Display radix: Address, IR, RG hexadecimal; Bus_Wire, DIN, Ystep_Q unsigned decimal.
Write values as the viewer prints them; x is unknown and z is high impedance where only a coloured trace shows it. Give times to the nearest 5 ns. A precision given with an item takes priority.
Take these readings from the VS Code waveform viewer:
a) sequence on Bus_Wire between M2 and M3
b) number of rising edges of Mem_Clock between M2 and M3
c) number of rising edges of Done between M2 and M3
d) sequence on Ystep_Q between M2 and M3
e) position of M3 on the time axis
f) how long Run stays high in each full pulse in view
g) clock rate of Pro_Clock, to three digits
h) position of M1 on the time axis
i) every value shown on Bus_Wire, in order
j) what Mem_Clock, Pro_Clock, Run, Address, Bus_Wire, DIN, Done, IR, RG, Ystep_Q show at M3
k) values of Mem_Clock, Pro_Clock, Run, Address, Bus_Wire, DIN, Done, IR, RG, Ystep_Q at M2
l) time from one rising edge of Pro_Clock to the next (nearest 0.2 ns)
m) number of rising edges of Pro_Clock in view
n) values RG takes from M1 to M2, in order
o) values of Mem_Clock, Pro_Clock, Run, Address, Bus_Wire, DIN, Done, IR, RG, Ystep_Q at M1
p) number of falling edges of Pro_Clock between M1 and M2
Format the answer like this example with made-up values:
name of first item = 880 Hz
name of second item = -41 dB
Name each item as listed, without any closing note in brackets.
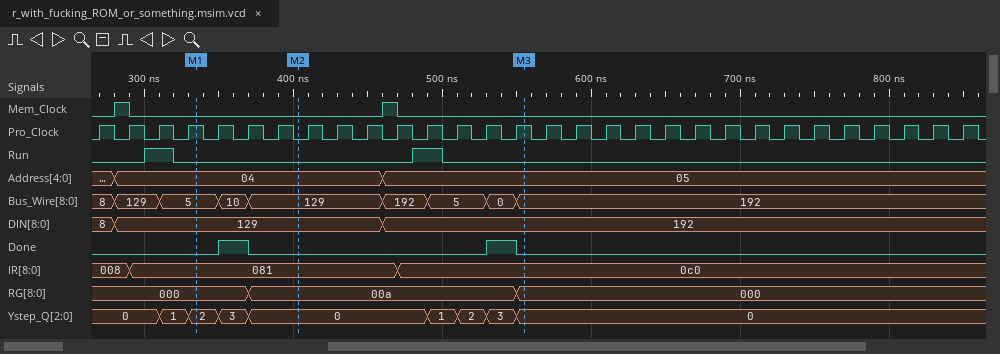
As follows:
sequence on Bus_Wire between M2 and M3 = 129, 192, 5, 0, 192
number of rising edges of Mem_Clock between M2 and M3 = 1
number of rising edges of Done between M2 and M3 = 1
sequence on Ystep_Q between M2 and M3 = 0, 1, 2, 3, 0
position of M3 on the time axis = 555 ns
how long Run stays high in each full pulse in view = 20 ns, 20 ns
clock rate of Pro_Clock, to three digits = 50.0 MHz
position of M1 on the time axis = 335 ns
every value shown on Bus_Wire, in order = 8, 129, 5, 10, 129, 192, 5, 0, 192
what Mem_Clock, Pro_Clock, Run, Address, Bus_Wire, DIN, Done, IR, RG, Ystep_Q show at M3 = Mem_Clock=0, Pro_Clock=1, Run=0, Address=05, Bus_Wire=192, DIN=192, Done=0, IR=0c0, RG=000, Ystep_Q=0
values of Mem_Clock, Pro_Clock, Run, Address, Bus_Wire, DIN, Done, IR, RG, Ystep_Q at M2 = Mem_Clock=0, Pro_Clock=0, Run=0, Address=04, Bus_Wire=129, DIN=129, Done=0, IR=081, RG=00a, Ystep_Q=0
time from one rising edge of Pro_Clock to the next = 20 ns
number of rising edges of Pro_Clock in view = 30
values RG takes from M1 to M2, in order = 000, 00a
values of Mem_Clock, Pro_Clock, Run, Address, Bus_Wire, DIN, Done, IR, RG, Ystep_Q at M1 = Mem_Clock=0, Pro_Clock=1, Run=0, Address=04, Bus_Wire=5, DIN=129, Done=0, IR=081, RG=000, Ystep_Q=2
number of falling edges of Pro_Clock between M1 and M2 = 4
